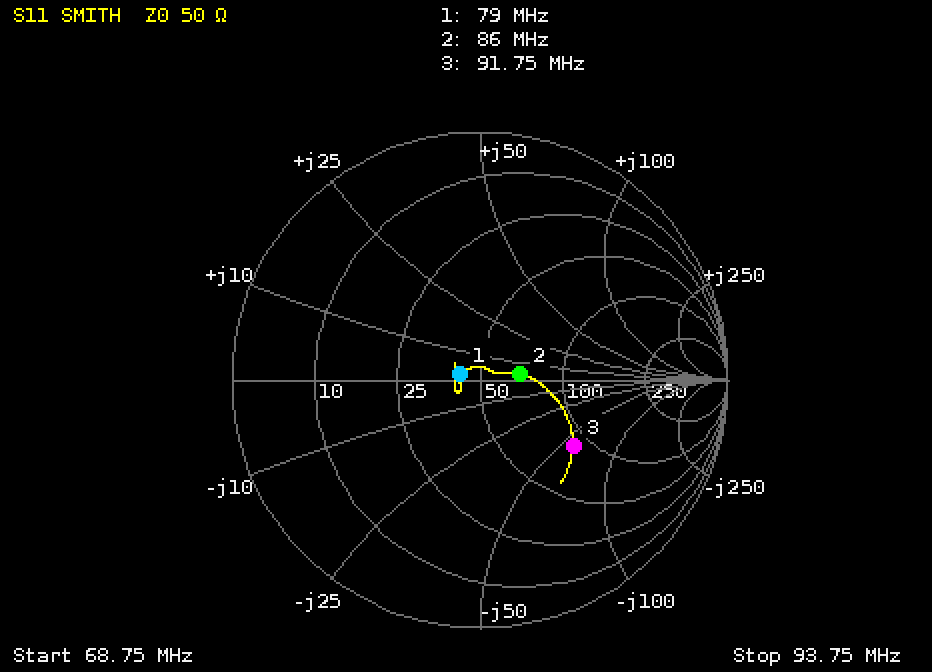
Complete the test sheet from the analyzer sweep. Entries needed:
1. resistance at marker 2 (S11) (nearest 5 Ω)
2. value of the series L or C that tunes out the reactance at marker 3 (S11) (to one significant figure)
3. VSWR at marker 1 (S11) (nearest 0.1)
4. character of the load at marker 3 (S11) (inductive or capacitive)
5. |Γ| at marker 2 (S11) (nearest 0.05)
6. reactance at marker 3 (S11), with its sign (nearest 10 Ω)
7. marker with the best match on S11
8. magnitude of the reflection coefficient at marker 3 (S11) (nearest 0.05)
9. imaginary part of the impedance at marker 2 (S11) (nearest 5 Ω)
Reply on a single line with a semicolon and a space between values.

70 Ω; 100 nH; 1.2; capacitive; 0.15; -60 Ω; marker 1; 0.45; +5 Ω
